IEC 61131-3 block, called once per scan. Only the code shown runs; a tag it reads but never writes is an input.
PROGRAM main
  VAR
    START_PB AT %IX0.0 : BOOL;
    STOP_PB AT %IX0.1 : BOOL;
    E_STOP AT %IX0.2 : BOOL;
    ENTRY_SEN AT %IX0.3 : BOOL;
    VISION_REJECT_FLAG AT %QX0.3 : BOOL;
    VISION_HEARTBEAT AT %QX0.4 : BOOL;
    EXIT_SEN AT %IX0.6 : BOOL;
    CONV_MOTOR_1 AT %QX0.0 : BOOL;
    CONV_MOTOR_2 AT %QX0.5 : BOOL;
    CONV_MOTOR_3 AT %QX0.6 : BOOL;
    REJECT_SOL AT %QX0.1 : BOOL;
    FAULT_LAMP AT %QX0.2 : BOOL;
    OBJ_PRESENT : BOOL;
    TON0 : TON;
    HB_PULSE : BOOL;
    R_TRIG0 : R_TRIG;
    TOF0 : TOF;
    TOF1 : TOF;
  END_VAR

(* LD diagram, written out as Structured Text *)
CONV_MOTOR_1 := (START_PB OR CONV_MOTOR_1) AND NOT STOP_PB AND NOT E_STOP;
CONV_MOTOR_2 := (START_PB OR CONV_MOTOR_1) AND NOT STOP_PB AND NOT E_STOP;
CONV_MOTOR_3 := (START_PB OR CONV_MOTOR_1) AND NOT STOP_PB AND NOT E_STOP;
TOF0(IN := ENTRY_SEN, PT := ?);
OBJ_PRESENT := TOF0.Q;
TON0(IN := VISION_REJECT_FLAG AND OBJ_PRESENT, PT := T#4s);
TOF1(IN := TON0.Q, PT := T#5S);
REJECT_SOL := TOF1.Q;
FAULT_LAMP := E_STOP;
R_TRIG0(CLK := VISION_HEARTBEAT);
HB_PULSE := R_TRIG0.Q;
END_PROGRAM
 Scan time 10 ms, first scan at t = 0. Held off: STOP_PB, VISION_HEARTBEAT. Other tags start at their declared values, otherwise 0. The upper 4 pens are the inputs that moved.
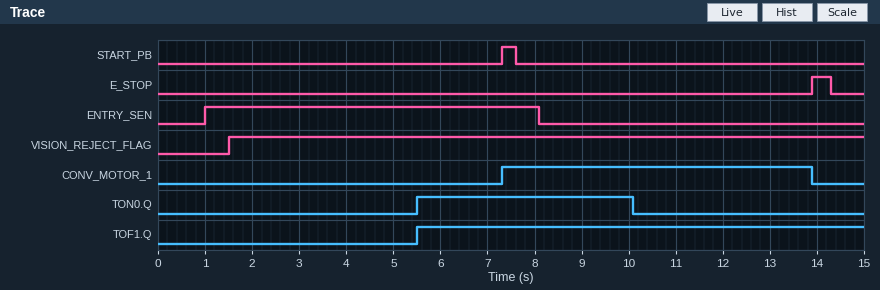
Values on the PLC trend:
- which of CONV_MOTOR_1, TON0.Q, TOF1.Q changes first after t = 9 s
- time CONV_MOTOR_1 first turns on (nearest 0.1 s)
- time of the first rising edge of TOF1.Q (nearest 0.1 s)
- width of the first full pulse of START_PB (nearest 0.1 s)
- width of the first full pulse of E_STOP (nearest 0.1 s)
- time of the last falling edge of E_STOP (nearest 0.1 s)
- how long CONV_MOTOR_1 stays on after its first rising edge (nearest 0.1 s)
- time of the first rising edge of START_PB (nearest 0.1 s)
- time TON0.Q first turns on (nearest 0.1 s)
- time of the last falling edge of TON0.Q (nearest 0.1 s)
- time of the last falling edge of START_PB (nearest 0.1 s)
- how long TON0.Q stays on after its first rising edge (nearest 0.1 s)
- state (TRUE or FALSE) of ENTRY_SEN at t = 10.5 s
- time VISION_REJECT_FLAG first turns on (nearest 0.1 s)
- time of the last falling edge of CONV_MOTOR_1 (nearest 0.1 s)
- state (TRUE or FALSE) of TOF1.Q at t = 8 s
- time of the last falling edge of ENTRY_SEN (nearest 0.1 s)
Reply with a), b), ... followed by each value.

a) TON0.Q
b) 7.3 s
c) 5.5 s
d) 0.3 s
e) 0.4 s
f) 14.3 s
g) 6.6 s
h) 7.3 s
i) 5.5 s
j) 10.1 s
k) 7.6 s
l) 4.6 s
m) FALSE
n) 1.5 s
o) 13.9 s
p) TRUE
q) 8.1 s
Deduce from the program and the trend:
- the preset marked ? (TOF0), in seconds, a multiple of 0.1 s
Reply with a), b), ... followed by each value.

a) 2.0 s
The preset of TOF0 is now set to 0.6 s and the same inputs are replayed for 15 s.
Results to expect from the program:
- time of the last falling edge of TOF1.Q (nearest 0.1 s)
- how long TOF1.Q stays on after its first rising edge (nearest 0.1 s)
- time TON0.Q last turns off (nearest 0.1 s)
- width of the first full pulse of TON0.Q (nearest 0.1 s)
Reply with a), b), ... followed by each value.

a) 13.7 s
b) 8.2 s
c) 8.7 s
d) 3.2 s
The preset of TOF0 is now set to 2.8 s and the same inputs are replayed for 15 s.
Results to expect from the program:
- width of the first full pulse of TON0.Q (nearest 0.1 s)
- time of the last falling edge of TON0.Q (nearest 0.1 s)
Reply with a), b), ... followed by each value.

a) 5.4 s
b) 10.9 s
